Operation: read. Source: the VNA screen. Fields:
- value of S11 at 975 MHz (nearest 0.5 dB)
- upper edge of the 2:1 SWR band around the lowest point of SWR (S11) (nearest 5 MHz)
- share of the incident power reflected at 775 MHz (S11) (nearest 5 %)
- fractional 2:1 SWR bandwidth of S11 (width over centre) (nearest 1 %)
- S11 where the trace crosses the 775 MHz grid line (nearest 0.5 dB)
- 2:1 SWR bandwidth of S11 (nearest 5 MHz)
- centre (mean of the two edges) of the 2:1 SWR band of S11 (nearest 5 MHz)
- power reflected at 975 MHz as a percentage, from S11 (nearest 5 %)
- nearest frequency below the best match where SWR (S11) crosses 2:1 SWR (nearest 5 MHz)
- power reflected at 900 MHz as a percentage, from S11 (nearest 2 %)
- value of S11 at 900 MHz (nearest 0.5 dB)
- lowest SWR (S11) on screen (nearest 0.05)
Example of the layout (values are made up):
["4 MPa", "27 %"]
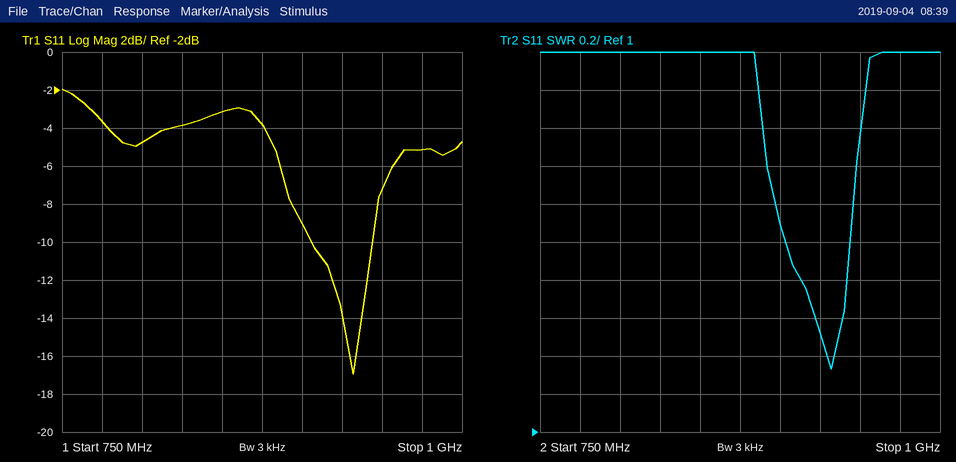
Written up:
["-5.0 dB", "945 MHz", "45 %", "4 %", "-3.5 dB", "40 MHz", "925 MHz", "30 %", "905 MHz", "12 %", "-9.0 dB", "1.35"]
